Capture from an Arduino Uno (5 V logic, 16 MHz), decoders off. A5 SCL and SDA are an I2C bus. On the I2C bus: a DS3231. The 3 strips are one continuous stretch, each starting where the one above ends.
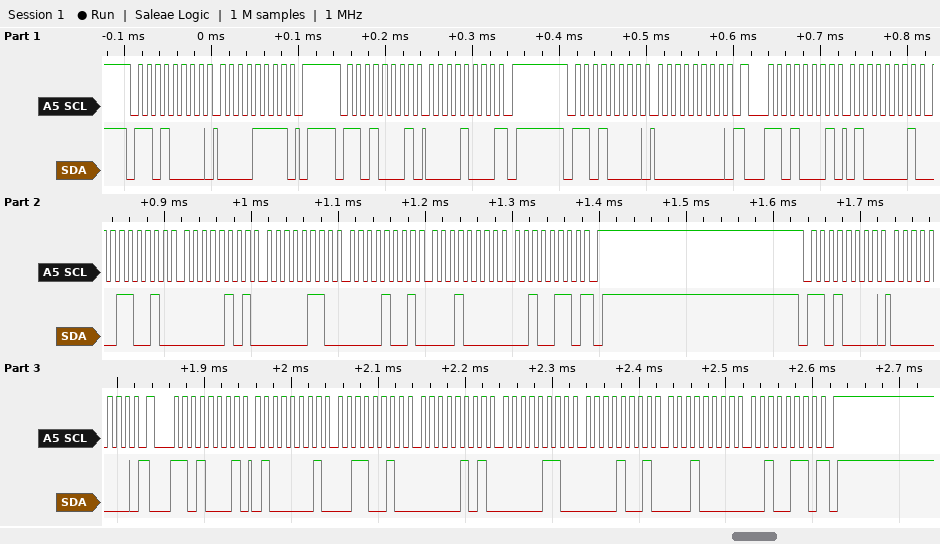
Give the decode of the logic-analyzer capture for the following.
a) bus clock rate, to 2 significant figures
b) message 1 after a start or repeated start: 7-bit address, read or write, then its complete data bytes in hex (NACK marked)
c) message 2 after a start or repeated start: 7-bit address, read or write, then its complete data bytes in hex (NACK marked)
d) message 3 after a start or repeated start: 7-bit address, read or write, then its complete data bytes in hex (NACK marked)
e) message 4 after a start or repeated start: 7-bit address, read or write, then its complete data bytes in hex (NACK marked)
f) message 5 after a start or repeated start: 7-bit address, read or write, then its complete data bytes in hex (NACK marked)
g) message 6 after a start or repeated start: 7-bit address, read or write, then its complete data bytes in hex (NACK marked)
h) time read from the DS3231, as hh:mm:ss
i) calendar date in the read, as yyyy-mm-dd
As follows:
100 kHz
0x68 write: 0F
0x68 read: 08 NACK
0x68 write: 00
0x68 read: 41 32 05 06 09 10 26 NACK
0x68 write: 00
0x68 read: 41 32 05 06 09 10 26 NACK
05:32:41
2026-10-09
